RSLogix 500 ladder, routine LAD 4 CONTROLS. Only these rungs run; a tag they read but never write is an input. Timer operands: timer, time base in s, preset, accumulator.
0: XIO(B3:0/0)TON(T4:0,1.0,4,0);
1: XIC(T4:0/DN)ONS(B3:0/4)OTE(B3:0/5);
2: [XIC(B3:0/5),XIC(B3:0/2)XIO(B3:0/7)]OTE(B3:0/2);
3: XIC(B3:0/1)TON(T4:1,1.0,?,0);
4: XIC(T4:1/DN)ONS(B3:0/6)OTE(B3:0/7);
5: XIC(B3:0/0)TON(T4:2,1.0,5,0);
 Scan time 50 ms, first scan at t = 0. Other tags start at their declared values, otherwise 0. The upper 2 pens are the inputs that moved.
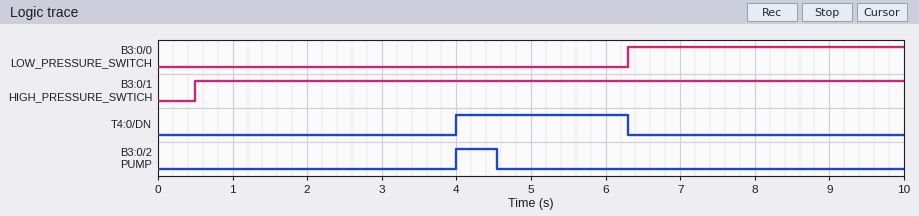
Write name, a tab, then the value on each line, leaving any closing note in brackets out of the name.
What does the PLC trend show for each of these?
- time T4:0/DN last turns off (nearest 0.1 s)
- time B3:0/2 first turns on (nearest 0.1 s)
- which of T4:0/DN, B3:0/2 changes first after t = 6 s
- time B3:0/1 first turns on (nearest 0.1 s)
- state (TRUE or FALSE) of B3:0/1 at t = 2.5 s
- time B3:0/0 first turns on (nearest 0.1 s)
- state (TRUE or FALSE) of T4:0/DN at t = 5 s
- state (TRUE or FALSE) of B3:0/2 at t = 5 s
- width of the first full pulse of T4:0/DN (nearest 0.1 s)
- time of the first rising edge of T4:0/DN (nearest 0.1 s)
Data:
time T4:0/DN last turns off	6.3 s
time B3:0/2 first turns on	4.0 s
which of T4:0/DN, B3:0/2 changes first after t = 6 s	T4:0/DN
time B3:0/1 first turns on	0.5 s
state (TRUE or FALSE) of B3:0/1 at t = 2.5 s	TRUE
time B3:0/0 first turns on	6.3 s
state (TRUE or FALSE) of T4:0/DN at t = 5 s	TRUE
state (TRUE or FALSE) of B3:0/2 at t = 5 s	FALSE
width of the first full pulse of T4:0/DN	2.3 s
time of the first rising edge of T4:0/DN	4.0 s
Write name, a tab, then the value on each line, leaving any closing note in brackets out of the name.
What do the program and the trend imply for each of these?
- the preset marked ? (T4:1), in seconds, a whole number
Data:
the preset marked ? (T4:1), in seconds, a whole number	4 s
